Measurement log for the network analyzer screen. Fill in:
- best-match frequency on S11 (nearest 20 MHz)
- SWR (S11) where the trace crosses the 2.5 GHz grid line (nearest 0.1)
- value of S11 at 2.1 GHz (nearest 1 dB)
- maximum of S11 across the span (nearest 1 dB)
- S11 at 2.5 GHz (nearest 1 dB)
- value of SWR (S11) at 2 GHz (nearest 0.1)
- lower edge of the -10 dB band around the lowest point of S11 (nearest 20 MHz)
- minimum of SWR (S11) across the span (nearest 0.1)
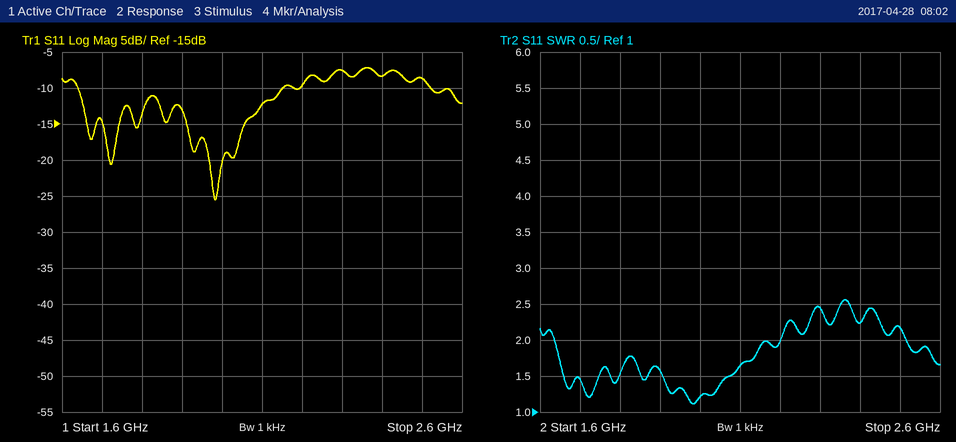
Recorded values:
1.98 GHz
2.2
-12 dB
-7 dB
-9 dB
1.2
1.64 GHz
1.1
